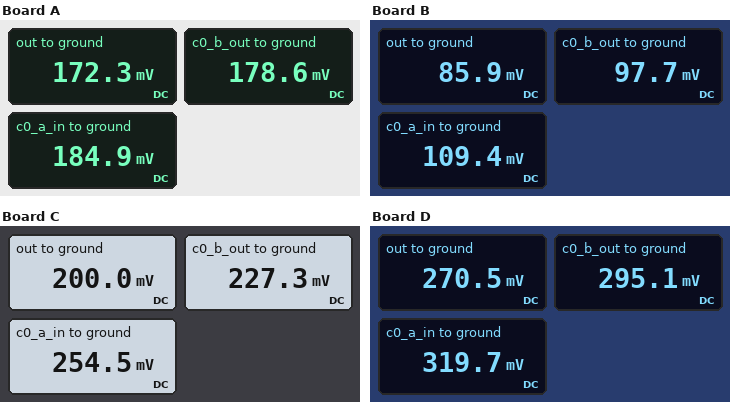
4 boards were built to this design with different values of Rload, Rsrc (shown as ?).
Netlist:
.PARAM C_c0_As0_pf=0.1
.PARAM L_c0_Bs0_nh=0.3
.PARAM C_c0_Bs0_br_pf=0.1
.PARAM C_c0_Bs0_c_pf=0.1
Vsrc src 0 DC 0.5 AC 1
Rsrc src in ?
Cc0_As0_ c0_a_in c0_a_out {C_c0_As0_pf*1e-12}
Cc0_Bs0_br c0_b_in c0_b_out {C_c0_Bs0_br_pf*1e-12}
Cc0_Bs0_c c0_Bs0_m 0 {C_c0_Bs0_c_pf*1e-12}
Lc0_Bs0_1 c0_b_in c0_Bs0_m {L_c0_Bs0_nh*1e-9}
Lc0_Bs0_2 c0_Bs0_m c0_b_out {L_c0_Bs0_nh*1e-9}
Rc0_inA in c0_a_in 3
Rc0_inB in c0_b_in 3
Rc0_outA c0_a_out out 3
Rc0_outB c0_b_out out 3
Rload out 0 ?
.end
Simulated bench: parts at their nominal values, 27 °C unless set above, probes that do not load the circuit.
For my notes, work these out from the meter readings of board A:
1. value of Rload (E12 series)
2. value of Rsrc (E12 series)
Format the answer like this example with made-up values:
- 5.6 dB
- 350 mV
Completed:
- 82 Ω
- 150 Ω
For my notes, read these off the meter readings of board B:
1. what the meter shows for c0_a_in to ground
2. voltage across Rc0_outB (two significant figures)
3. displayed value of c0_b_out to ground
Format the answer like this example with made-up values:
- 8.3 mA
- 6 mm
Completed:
- 109.4 mV
- 12 mV
- 97.7 mV
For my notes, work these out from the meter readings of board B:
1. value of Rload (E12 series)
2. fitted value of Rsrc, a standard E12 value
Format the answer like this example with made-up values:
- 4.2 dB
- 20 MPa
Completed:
- 22 Ω
- 100 Ω
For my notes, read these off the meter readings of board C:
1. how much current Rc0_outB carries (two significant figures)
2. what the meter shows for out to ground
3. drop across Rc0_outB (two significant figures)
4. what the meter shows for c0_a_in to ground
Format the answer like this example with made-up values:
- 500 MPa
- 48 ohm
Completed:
- 9.1 mA
- 200.0 mV
- 27 mV
- 254.5 mV
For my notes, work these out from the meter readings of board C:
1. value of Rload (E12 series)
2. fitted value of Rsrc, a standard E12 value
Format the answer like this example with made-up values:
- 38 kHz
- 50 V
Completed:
- 22 Ω
- 27 Ω
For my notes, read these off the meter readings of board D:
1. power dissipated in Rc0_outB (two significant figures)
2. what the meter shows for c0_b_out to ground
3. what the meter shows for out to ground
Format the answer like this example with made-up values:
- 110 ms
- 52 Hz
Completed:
- 200 µW
- 295.1 mV
- 270.5 mV
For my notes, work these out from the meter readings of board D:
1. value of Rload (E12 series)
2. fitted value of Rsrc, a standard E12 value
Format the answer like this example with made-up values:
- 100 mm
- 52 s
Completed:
- 33 Ω
- 22 Ω
